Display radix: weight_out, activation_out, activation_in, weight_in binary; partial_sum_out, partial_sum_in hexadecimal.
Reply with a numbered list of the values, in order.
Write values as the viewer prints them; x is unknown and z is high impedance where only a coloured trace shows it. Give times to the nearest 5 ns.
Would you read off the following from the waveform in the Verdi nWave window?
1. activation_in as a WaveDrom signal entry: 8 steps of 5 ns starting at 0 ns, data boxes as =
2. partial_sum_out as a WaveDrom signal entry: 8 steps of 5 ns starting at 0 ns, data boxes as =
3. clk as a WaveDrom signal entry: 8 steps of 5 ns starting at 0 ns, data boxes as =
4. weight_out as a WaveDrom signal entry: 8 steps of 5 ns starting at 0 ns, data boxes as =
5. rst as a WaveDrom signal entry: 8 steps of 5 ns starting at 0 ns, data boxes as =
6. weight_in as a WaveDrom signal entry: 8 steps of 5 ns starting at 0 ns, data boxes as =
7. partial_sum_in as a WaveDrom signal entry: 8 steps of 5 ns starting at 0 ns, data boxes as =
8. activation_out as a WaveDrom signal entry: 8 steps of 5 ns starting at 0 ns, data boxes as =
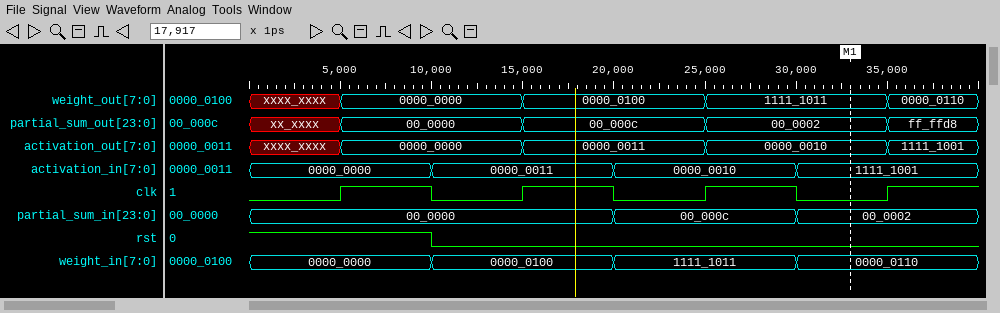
1. {name: 'activation_in', wave: '=.=.=.=.', data: '0000_0000 0000_0011 0000_0010 1111_1001'}
2. {name: 'partial_sum_out', wave: 'x=.=.=.=', data: '00_0000 00_000c 00_0002 ff_ffd8'}
3. {name: 'clk', wave: '01010101'}
4. {name: 'weight_out', wave: 'x=.=.=.=', data: '0000_0000 0000_0100 1111_1011 0000_0110'}
5. {name: 'rst', wave: '1.0.....'}
6. {name: 'weight_in', wave: '=.=.=.=.', data: '0000_0000 0000_0100 1111_1011 0000_0110'}
7. {name: 'partial_sum_in', wave: '=...=.=.', data: '00_0000 00_000c 00_0002'}
8. {name: 'activation_out', wave: 'x=.=.=.=', data: '0000_0000 0000_0011 0000_0010 1111_1001'}
